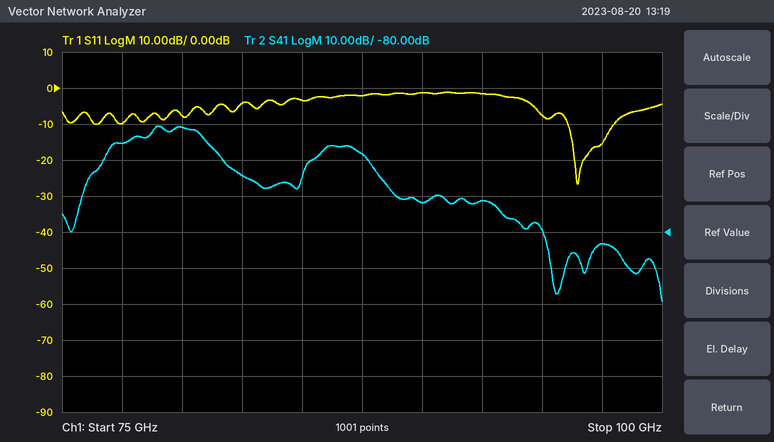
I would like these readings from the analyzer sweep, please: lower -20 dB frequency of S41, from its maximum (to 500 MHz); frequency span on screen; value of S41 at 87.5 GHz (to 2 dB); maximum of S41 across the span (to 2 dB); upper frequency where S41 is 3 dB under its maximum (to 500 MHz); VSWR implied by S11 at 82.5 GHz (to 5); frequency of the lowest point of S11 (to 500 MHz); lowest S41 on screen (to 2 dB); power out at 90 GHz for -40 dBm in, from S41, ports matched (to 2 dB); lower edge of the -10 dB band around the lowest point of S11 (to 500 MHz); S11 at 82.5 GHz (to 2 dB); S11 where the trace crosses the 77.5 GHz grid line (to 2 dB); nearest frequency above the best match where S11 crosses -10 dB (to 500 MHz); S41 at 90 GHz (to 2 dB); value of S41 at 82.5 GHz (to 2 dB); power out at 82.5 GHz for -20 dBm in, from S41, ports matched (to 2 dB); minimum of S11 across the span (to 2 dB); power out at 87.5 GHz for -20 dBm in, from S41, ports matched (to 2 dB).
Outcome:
76.0 GHz
25 GHz
-58 dB
-50 dB
81.0 GHz
5
96.5 GHz
-100 dB
-112 dBm
96.0 GHz
-4 dB
-10 dB
98.0 GHz
-72 dB
-64 dB
-84 dBm
-26 dB
-78 dBm
